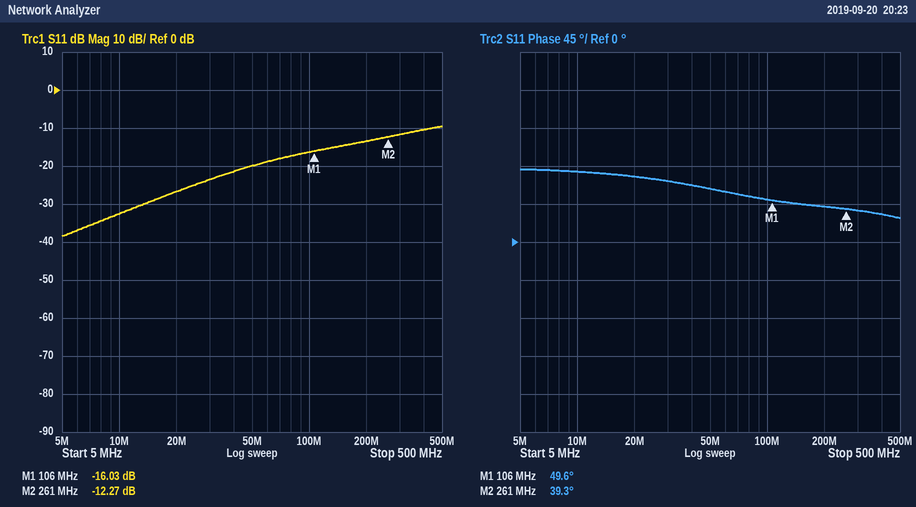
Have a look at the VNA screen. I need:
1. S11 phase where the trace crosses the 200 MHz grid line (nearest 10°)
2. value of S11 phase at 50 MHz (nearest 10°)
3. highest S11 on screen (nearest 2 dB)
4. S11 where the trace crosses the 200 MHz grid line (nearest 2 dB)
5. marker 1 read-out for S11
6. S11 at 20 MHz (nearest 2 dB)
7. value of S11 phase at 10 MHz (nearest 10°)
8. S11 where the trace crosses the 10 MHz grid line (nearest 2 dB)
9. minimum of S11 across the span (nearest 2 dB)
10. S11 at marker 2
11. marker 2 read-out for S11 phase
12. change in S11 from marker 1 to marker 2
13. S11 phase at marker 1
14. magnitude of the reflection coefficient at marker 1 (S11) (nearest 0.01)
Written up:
40°
60°
-10 dB
-14 dB
-16.03 dB
-26 dB
80°
-32 dB
-38 dB
-12.27 dB
39.3°
3.76 dB
49.6°
0.16
